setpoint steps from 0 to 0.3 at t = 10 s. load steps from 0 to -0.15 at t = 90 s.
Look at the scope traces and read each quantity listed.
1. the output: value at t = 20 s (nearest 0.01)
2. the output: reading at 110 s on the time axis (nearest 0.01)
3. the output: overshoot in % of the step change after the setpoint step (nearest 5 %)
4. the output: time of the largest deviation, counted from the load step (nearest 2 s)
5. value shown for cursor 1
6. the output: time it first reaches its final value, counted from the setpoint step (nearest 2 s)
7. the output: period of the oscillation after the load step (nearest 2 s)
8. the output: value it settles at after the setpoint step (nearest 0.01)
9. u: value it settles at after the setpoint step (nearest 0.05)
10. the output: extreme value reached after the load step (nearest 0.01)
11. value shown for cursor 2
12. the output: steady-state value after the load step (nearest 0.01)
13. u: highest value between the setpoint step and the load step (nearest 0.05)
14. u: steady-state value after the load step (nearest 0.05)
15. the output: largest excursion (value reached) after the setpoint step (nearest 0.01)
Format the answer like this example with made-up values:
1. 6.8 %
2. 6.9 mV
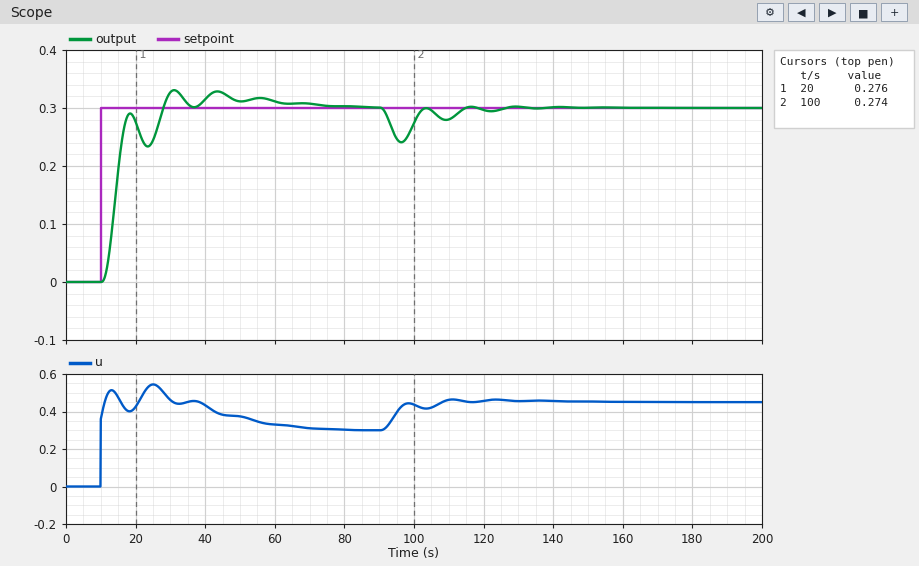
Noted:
1. 0.28
2. 0.28
3. 10 %
4. 6 s
5. 0.276
6. 18 s
7. 12 s
8. 0.30
9. 0.30
10. 0.24
11. 0.274
12. 0.30
13. 0.55
14. 0.45
15. 0.33
